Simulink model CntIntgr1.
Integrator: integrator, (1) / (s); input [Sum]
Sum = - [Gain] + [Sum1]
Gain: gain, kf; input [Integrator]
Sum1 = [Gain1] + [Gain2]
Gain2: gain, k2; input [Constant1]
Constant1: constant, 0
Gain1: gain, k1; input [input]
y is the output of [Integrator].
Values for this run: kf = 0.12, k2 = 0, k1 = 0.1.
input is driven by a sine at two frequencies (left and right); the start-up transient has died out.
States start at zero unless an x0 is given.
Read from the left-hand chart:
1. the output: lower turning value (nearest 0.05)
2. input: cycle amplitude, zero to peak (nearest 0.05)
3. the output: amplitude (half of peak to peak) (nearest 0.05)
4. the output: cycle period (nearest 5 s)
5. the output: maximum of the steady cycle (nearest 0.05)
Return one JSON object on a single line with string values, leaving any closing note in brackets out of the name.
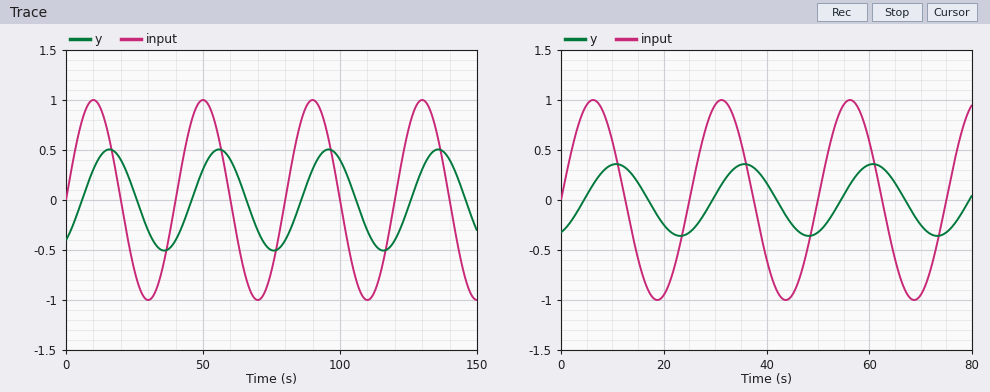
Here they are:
{"the output: lower turning value": "-0.50", "input: cycle amplitude, zero to peak": "1.00", "the output: amplitude (half of peak to peak)": "0.50", "the output: cycle period": "40 s", "the output: maximum of the steady cycle": "0.50"}
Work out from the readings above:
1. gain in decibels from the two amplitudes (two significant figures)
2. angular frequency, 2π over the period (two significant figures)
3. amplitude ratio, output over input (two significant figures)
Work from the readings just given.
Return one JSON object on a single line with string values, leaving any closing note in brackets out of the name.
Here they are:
{"gain in decibels from the two amplitudes": "-6.0 dB", "angular frequency, 2π over the period": "0.16 rad/s", "amplitude ratio, output over input": "0.50"}
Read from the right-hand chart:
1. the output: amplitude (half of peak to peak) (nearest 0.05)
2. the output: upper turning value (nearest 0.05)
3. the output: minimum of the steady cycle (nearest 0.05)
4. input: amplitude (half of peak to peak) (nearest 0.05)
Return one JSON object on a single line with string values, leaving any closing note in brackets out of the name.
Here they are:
{"the output: amplitude (half of peak to peak)": "0.35", "the output: upper turning value": "0.35", "the output: minimum of the steady cycle": "-0.35", "input: amplitude (half of peak to peak)": "1.00"}
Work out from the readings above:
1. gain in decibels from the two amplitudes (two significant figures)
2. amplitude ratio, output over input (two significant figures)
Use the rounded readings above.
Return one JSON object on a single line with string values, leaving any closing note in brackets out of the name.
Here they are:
{"gain in decibels from the two amplitudes": "-9.1 dB", "amplitude ratio, output over input": "0.35"}
